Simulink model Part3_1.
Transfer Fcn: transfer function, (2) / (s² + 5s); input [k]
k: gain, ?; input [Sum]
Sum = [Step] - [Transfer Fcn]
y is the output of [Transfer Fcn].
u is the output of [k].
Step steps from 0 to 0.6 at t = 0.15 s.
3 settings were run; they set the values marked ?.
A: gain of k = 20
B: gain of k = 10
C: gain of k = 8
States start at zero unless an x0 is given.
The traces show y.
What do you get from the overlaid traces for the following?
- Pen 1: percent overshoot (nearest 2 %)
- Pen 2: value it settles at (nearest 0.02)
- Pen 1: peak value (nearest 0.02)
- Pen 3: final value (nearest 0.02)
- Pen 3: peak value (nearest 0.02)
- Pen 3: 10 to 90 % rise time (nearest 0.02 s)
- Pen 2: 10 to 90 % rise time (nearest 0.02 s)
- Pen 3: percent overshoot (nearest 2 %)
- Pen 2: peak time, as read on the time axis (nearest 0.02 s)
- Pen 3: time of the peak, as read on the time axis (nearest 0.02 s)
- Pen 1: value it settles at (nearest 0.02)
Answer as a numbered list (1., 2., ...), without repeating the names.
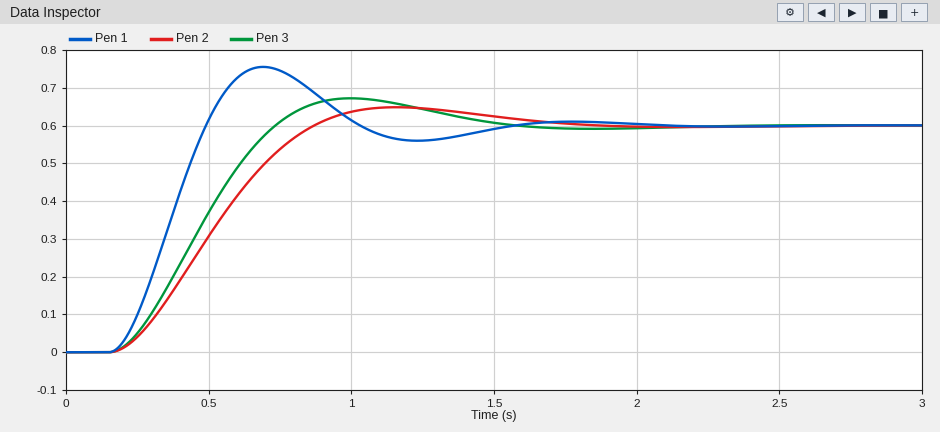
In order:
1. 26 %
2. 0.60
3. 0.76
4. 0.60
5. 0.68
6. 0.40 s
7. 0.48 s
8. 12 %
9. 1.16 s
10. 1.00 s
11. 0.60
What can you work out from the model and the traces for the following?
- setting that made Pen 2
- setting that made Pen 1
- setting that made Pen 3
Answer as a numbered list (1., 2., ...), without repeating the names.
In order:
1. C
2. A
3. B
